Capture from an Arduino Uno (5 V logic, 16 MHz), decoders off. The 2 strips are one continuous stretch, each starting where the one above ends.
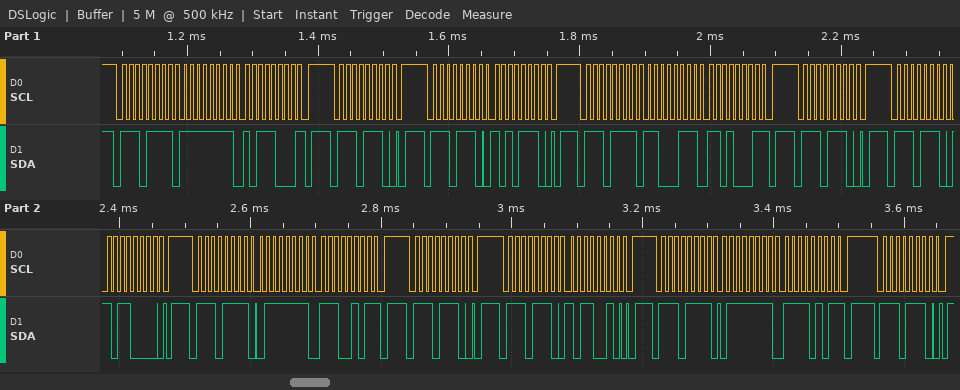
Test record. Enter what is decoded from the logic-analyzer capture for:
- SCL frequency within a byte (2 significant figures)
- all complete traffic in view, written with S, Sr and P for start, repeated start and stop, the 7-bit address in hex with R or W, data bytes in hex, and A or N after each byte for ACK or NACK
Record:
100 kHz
S 77R A FF A B8 N P S 77W A P S 77W A AE A P S 77R A C7 A D1 N P S 77W A P S 77W A B0 A P S 77R A 7F A E5 N P S 77W A P S 77W A B2 A P S 77R A 7F A F5 N P S 77W A P
